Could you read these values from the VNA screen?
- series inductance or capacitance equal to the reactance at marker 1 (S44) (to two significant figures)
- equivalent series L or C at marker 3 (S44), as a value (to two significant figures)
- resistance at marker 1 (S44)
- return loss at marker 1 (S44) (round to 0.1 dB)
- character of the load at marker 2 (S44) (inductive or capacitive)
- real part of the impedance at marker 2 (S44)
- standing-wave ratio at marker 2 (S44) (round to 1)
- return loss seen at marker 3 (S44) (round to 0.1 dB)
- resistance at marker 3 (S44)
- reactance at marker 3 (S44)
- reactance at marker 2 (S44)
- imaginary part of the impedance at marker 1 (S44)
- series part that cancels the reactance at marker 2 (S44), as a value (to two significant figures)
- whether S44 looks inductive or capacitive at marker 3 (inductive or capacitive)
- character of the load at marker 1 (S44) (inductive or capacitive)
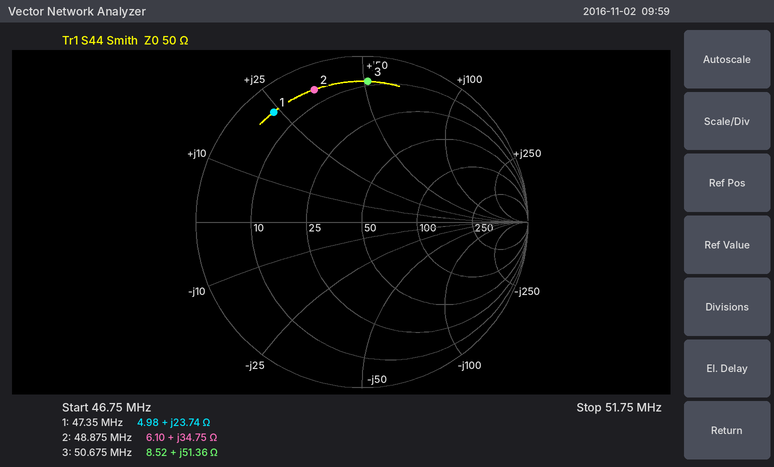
80 nH
160 nH
4.98 Ω
1.4 dB
inductive
6.10 Ω
12
1.4 dB
8.52 Ω
+51.36 Ω
+34.75 Ω
+23.74 Ω
94 pF
inductive
inductive
